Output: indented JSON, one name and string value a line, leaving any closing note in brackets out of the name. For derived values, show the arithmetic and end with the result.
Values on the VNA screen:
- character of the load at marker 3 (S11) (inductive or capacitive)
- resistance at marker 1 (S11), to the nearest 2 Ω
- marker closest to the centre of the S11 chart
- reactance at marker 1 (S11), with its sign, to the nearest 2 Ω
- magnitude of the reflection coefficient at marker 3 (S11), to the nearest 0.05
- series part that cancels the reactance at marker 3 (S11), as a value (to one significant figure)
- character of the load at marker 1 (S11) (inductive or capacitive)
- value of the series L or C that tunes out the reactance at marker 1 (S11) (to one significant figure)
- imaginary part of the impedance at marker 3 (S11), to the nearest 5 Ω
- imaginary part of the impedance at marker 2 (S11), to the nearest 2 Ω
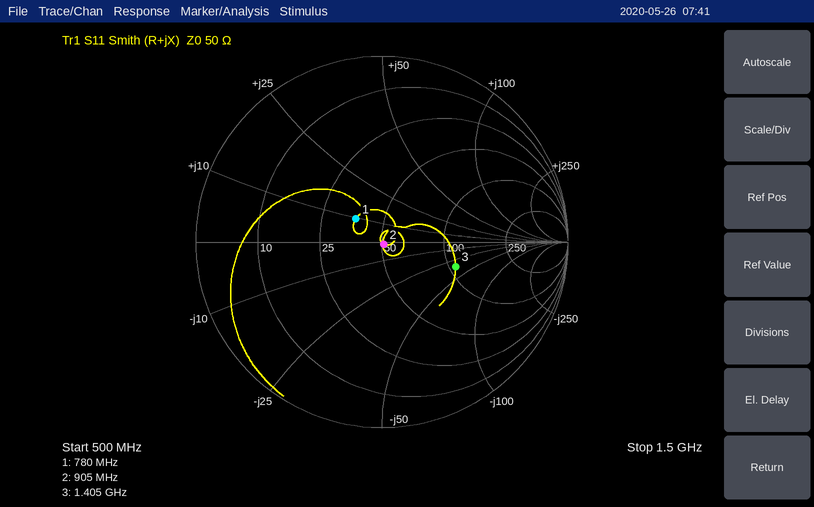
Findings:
{
  "character of the load at marker 3 (S11)": "capacitive",
  "resistance at marker 1 (S11), to the nearest 2 Ω": "36 Ω",
  "marker closest to the centre of the S11 chart": "marker 2",
  "reactance at marker 1 (S11), with its sign, to the nearest 2 Ω": "+10 Ω",
  "magnitude of the reflection coefficient at marker 3 (S11), to the nearest 0.05": "0.40",
  "series part that cancels the reactance at marker 3 (S11), as a value": "L = 35 Ω/(2π × 1.405 GHz) ≈ 4 nH",
  "character of the load at marker 1 (S11)": "inductive",
  "value of the series L or C that tunes out the reactance at marker 1 (S11)": "C = 1/(2π × 780 MHz × 10 Ω) ≈ 20 pF",
  "imaginary part of the impedance at marker 3 (S11), to the nearest 5 Ω": "-35 Ω",
  "imaginary part of the impedance at marker 2 (S11), to the nearest 2 Ω": "-2 Ω"
}
